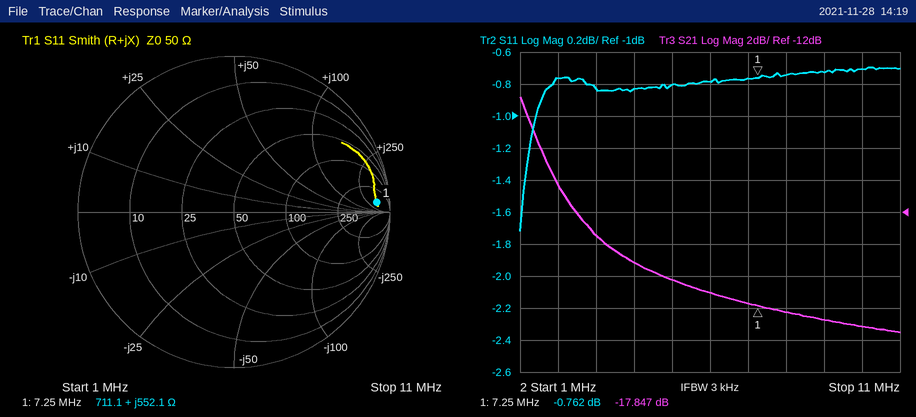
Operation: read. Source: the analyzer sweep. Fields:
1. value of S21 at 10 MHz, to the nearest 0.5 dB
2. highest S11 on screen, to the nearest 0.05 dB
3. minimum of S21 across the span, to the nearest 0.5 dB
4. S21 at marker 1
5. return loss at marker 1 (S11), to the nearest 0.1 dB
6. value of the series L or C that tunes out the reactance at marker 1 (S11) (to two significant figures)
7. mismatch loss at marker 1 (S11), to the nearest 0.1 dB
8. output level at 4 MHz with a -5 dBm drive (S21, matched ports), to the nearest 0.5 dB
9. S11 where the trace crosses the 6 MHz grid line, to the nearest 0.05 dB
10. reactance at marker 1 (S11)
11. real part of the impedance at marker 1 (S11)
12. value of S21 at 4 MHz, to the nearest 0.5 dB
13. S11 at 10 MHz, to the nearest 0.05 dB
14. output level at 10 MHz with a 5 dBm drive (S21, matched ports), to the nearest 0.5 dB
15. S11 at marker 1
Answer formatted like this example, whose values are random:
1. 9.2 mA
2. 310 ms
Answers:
1. -19.0 dB
2. -0.70 dB
3. -19.5 dB
4. -17.847 dB
5. 0.8 dB
6. 40 pF
7. 7.9 dB
8. -20.0 dBm
9. -0.80 dB
10. +552.1 Ω
11. 711.1 Ω
12. -15.0 dB
13. -0.70 dB
14. -14.0 dBm
15. -0.762 dB
